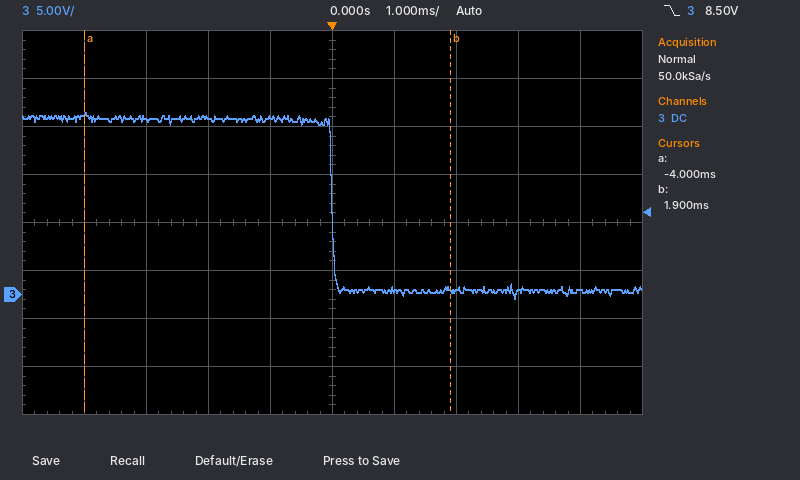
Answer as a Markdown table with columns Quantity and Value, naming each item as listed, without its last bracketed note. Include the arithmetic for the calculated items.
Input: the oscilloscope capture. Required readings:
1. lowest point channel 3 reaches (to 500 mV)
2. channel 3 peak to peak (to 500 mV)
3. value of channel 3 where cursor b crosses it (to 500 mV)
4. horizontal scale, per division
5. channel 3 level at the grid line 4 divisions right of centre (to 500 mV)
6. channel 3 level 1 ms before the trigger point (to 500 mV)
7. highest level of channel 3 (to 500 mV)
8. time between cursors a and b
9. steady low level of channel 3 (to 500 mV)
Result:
| Quantity | Value |
|---|---|
| lowest point channel 3 reaches | -500 mV |
| channel 3 peak to peak | 19.0 V − (-500 mV) = 19.5 V |
| value of channel 3 where cursor b crosses it | 500 mV |
| horizontal scale, per division | 1 ms |
| channel 3 level at the grid line 4 divisions right of centre | 500 mV |
| channel 3 level 1 ms before the trigger point | 18.5 V |
| highest level of channel 3 | 19.0 V |
| time between cursors a and b | 1.9 ms − (-4 ms) = 5.9 ms |
| steady low level of channel 3 | 500 mV |
